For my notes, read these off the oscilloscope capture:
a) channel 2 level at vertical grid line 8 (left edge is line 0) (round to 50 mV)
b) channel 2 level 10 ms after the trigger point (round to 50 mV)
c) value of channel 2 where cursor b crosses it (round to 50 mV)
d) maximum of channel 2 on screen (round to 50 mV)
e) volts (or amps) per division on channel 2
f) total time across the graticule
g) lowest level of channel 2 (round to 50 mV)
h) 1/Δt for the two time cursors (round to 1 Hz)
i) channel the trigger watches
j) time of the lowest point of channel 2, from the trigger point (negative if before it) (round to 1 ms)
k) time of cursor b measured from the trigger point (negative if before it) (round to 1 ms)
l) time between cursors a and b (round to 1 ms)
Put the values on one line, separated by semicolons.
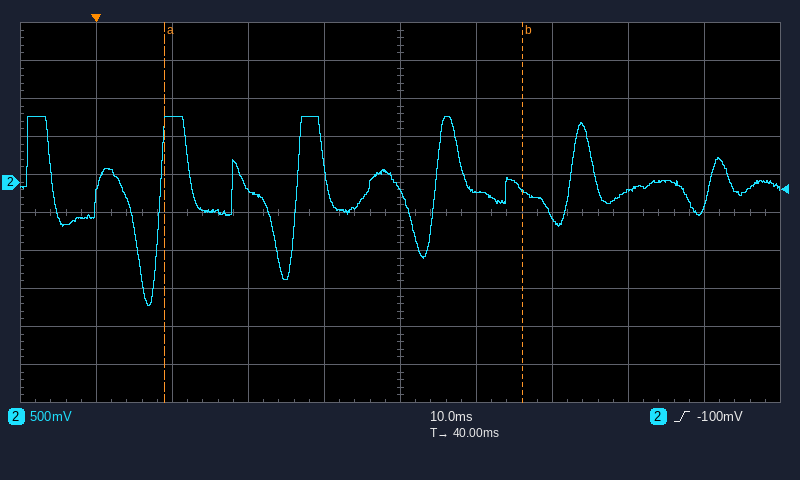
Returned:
-100 mV; 850 mV; -100 mV; 850 mV; 500 mV; 100 ms; -1.60 V; 21 Hz; channel 2; +7 ms; +56 ms; 47 ms
